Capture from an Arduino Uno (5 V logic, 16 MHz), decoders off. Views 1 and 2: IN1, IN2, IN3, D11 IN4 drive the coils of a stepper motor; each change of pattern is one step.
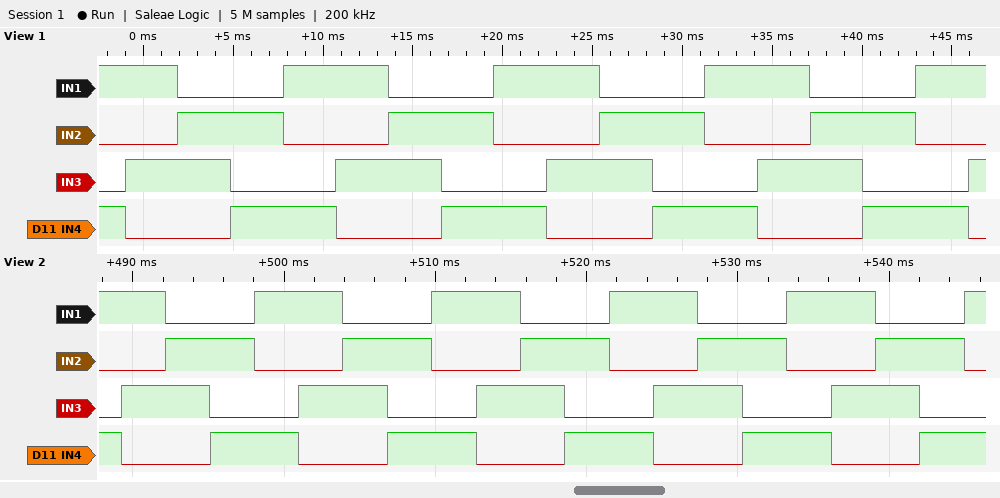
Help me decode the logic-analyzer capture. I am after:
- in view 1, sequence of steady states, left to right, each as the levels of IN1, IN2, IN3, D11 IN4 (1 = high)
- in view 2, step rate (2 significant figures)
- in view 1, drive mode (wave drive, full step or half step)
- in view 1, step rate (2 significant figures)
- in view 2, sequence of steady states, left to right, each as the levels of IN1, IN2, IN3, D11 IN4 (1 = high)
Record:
1001 1010 0110 0101 1001 1010 0110 0101 1001 1010 0110 0101 1001 1010 0110 0101 1001 1010
340 steps/s
full step
340 steps/s
1001 1010 0110 0101 1001 1010 0110 0101 1001 1010 0110 0101 1001 1010 0110 0101 1001 1010 0110 0101 1001
